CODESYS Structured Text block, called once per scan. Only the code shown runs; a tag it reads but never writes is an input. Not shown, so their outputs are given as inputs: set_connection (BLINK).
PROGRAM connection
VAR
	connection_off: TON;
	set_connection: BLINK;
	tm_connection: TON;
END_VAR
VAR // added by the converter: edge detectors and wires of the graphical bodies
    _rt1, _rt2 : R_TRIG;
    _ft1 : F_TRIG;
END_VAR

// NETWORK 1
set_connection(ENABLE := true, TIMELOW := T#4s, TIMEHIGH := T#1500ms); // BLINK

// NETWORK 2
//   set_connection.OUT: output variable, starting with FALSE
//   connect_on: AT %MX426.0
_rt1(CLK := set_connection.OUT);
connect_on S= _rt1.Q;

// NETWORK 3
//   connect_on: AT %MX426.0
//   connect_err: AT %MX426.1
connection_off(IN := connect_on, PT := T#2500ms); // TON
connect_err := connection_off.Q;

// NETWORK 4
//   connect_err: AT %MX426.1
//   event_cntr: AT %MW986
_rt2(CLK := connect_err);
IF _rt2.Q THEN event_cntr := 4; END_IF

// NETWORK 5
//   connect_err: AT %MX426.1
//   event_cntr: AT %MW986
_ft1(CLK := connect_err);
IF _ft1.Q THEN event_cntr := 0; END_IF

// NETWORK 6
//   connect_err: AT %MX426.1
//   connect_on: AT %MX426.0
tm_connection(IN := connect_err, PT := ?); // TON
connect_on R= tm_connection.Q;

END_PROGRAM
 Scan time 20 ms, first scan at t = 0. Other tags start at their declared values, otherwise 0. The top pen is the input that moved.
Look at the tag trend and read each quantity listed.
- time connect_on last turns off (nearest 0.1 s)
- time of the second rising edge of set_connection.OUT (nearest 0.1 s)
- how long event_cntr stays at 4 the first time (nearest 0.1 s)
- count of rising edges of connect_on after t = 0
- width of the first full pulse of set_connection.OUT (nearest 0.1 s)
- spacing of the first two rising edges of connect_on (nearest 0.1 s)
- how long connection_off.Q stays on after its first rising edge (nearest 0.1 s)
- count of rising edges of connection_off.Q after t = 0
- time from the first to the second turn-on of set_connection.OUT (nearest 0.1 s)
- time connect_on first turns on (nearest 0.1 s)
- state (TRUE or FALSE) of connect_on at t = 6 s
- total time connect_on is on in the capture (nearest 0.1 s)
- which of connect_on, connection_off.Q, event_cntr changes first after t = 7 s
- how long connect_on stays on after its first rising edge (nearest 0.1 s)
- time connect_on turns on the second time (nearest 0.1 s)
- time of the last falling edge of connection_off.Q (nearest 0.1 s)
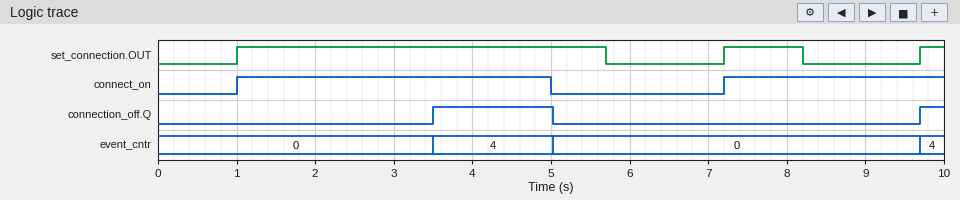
5.0 s
7.2 s
1.5 s
2
4.7 s
6.2 s
1.5 s
2
6.2 s
1.0 s
FALSE
6.8 s
connect_on
4.0 s
7.2 s
5.0 s
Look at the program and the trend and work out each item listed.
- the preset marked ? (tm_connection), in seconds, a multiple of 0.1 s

1.5 s
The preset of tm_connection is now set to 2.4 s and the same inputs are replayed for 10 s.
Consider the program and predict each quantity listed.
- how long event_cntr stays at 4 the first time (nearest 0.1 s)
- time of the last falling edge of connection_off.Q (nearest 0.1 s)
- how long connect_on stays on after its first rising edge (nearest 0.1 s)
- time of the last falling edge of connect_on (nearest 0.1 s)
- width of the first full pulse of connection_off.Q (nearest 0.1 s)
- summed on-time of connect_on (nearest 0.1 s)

2.4 s
5.9 s
4.9 s
5.9 s
2.4 s
7.7 s
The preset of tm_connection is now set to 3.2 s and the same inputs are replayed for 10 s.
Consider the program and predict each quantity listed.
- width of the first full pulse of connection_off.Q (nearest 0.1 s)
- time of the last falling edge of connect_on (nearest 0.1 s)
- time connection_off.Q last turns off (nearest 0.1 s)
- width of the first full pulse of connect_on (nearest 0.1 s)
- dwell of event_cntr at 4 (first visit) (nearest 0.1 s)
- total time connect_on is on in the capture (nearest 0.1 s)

3.2 s
6.7 s
6.7 s
5.7 s
3.2 s
8.5 s
